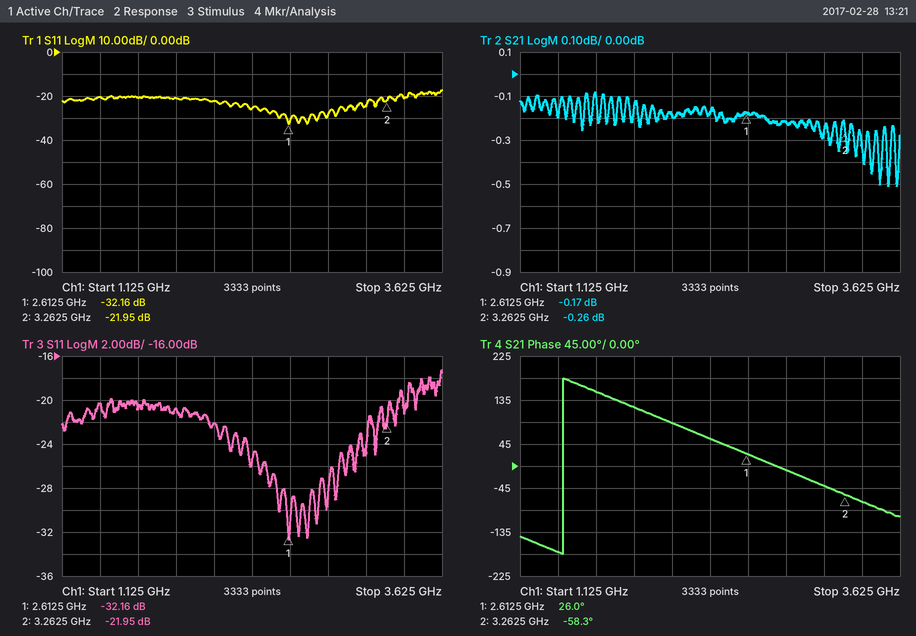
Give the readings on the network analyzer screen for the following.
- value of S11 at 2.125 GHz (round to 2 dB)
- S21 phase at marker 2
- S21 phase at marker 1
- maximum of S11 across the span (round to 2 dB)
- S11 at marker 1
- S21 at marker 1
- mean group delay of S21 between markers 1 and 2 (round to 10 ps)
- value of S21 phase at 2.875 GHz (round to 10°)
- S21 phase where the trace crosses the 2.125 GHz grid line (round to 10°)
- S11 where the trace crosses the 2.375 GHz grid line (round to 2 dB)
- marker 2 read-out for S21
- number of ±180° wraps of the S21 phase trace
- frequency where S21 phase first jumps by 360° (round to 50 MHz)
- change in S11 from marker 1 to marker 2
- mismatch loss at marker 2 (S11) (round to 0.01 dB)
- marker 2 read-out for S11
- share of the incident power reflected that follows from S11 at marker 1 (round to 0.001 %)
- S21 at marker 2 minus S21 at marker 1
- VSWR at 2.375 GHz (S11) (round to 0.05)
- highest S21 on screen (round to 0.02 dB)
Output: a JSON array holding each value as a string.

["-22 dB", "-58.3°", "26.0°", "-18 dB", "-32.16 dB", "-0.17 dB", "360 ps", "-10°", "90°", "-26 dB", "-0.26 dB", "1", "1.40 GHz", "10.21 dB", "0.03 dB", "-21.95 dB", "0.061 %", "-0.09 dB", "1.10", "-0.08 dB"]
